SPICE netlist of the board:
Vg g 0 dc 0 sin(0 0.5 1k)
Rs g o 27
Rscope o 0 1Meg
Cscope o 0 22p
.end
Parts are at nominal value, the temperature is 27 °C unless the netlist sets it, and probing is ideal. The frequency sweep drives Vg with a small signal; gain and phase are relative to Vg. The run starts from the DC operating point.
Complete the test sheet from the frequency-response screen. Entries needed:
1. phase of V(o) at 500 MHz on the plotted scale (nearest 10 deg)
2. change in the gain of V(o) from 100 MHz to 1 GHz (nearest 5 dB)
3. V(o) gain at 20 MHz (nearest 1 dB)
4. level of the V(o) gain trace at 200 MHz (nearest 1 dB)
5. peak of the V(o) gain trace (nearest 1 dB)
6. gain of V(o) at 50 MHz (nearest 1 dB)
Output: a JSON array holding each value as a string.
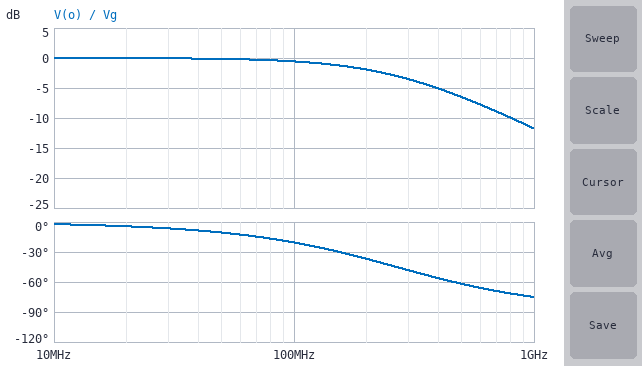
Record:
["-60 deg", "-10 dB", "0 dB", "-2 dB", "0 dB", "0 dB"]
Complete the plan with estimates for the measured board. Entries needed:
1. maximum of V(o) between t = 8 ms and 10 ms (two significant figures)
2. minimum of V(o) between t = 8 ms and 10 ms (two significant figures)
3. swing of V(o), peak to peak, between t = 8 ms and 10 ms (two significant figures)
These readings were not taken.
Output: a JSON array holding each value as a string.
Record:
["500 mV", "-500 mV", "1.0 V"]
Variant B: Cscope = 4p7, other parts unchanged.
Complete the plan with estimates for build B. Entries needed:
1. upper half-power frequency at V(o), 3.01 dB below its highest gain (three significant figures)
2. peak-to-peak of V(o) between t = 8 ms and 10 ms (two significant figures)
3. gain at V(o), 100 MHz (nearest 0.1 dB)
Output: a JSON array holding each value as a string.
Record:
["1.25 GHz", "1.0 V", "0 dB"]
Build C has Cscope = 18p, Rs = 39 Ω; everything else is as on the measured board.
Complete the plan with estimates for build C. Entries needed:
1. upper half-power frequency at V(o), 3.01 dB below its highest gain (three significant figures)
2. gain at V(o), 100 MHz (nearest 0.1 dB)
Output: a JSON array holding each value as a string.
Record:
["227 MHz", "-0.8 dB"]
